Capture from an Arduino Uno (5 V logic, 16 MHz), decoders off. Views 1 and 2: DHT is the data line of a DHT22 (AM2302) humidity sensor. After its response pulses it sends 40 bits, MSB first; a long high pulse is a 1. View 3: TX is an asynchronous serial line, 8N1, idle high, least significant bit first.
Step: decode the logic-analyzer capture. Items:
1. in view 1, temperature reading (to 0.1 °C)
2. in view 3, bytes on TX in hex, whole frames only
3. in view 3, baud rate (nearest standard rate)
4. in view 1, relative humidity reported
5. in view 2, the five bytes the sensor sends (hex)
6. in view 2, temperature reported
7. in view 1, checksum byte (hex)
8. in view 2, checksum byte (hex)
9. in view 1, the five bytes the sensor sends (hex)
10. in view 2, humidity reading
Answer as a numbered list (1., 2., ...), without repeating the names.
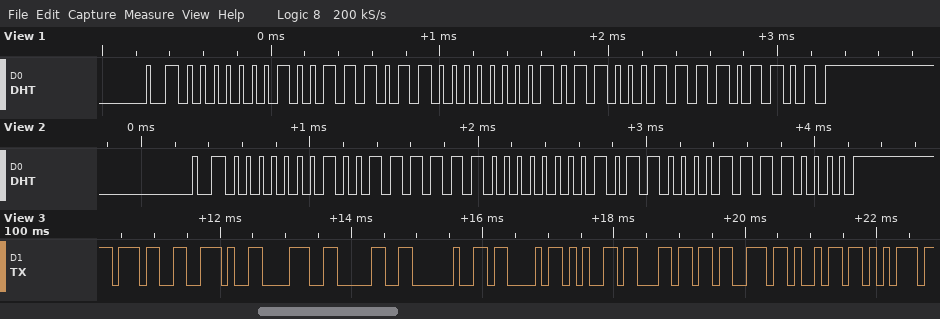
1. 17.7 °C
2. 37 2E 38 30 20 43 65 6C 73 69 75
3. 9600 baud
4. 31.5 %
5. 01 3F 00 B0 F0
6. 17.6 °C
7. 0xED
8. 0xF0
9. 01 3B 00 B1 ED
10. 31.9 %
